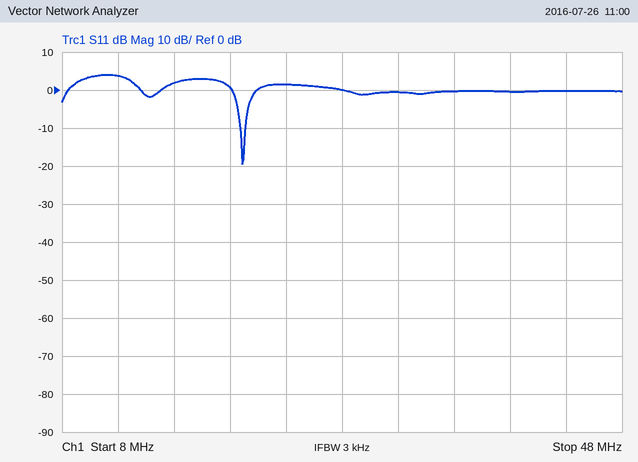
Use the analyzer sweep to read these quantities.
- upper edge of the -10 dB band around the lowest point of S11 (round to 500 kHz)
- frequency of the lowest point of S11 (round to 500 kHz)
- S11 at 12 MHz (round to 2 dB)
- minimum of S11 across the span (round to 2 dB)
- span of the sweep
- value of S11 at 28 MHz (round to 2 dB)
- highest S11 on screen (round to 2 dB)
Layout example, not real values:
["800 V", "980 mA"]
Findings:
["21.0 MHz", "21.0 MHz", "4 dB", "-20 dB", "40 MHz", "0 dB", "4 dB"]
